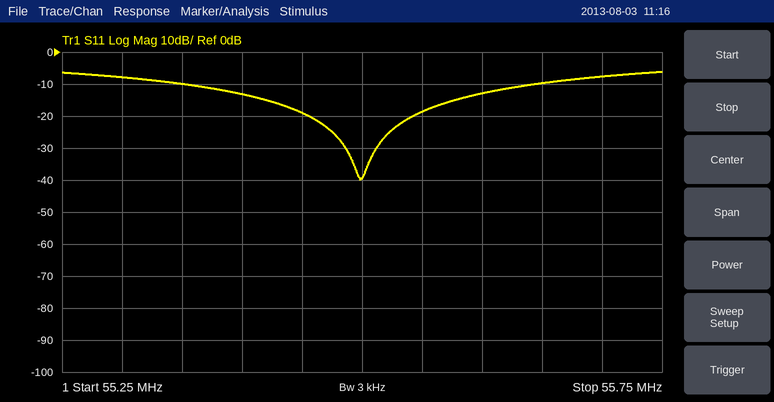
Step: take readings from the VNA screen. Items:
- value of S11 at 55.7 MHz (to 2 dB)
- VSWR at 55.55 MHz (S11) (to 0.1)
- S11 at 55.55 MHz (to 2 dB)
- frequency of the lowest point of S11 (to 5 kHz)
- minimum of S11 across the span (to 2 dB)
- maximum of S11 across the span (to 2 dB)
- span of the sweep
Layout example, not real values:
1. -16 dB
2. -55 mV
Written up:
1. -8 dB
2. 1.3
3. -18 dB
4. 55.500 MHz
5. -40 dB
6. -6 dB
7. 500 kHz
